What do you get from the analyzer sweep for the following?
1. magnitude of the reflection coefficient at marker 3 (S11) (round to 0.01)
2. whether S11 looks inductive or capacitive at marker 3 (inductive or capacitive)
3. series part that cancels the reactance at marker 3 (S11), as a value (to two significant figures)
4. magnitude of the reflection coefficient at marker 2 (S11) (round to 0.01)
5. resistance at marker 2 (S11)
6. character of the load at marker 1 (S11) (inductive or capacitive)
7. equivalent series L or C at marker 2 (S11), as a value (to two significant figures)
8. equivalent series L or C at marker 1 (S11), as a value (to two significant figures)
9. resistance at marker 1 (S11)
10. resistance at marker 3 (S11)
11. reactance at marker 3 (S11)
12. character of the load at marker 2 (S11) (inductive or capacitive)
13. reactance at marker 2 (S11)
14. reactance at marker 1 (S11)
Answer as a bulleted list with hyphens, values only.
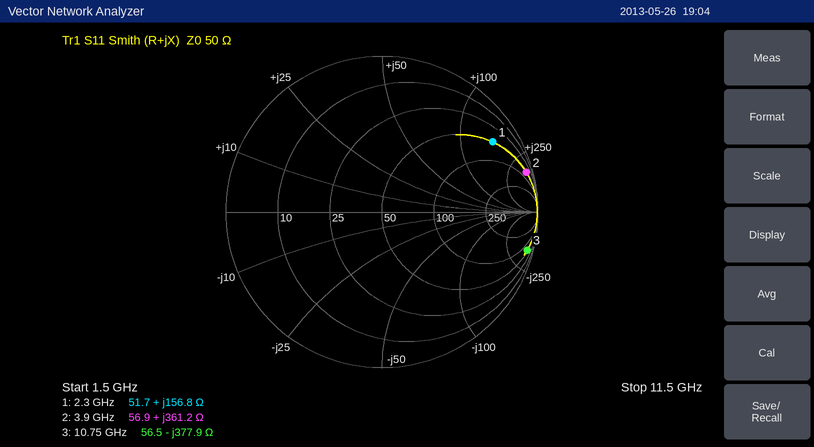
- 0.96
- capacitive
- 5.6 nH
- 0.96
- 56.9 Ω
- inductive
- 15 nH
- 11 nH
- 51.7 Ω
- 56.5 Ω
- -377.9 Ω
- inductive
- +361.2 Ω
- +156.8 Ω
